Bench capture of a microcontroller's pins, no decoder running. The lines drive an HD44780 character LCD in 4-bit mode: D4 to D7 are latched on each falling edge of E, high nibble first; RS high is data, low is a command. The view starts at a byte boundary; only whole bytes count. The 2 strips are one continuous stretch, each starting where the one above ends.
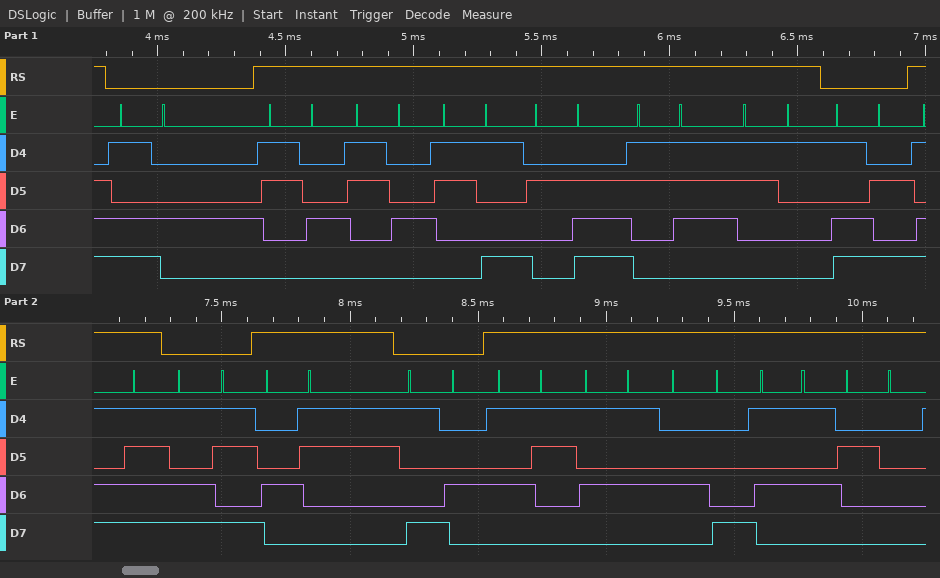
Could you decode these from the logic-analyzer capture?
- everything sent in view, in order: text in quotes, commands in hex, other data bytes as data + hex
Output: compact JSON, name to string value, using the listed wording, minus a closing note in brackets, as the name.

{"everything sent in view, in order: text in quotes, commands in hex, other data bytes as data + hex": "0xD4 \"449.71\" 0xDA data DF 0xDB \"C\" 0x94 \"SUHU \""}
